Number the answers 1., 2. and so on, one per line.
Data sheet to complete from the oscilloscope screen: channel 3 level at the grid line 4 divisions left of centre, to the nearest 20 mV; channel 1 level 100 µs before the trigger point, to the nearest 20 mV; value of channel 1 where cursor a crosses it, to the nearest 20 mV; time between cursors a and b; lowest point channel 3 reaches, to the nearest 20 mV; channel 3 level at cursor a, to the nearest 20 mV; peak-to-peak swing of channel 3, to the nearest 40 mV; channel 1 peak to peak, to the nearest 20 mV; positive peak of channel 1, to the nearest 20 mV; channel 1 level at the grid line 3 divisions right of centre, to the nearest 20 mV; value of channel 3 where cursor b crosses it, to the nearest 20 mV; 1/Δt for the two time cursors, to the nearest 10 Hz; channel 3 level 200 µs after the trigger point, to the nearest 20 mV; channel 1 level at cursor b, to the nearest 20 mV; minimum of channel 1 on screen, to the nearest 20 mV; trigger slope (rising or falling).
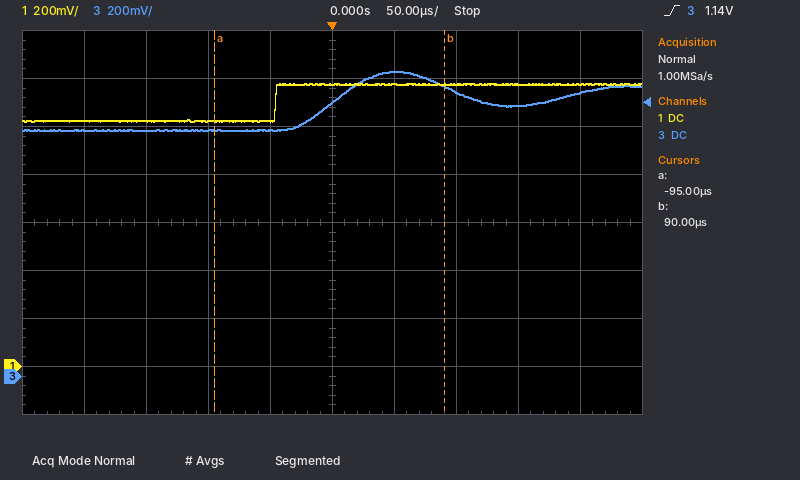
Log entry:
1. 1.02 V
2. 1.02 V
3. 1.02 V
4. 185 µs
5. 1.02 V
6. 1.02 V
7. 240 mV
8. 160 mV
9. 1.18 V
10. 1.18 V
11. 1.20 V
12. 5.41 kHz
13. 1.18 V
14. 1.18 V
15. 1.02 V
16. rising
